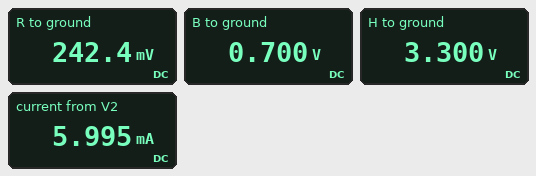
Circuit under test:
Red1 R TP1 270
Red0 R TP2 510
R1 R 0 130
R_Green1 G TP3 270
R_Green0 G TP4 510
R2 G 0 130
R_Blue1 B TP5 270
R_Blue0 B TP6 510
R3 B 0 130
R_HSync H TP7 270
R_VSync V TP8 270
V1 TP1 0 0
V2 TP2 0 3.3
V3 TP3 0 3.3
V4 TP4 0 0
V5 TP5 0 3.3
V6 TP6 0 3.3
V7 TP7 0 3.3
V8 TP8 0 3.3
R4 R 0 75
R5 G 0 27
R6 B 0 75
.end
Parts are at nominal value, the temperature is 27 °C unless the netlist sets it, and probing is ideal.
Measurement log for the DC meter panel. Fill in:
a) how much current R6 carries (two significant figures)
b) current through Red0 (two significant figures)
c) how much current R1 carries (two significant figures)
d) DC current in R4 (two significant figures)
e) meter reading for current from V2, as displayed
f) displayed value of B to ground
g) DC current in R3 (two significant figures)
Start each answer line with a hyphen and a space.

- 9.3 mA
- 6.0 mA
- 1.9 mA
- 3.2 mA
- 5.995 mA
- 0.700 V
- 5.4 mA
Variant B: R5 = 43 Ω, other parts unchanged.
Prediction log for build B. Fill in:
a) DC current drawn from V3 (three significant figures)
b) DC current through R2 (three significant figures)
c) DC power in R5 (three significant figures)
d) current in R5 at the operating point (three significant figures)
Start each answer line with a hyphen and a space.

- 11.0 mA
- 2.57 mA
- 2.59 mW
- 7.76 mA
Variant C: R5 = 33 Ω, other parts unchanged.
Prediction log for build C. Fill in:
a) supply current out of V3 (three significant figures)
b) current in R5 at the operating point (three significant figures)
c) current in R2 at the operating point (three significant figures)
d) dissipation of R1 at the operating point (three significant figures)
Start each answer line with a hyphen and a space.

- 11.2 mA
- 8.48 mA
- 2.15 mA
- 452 µW
